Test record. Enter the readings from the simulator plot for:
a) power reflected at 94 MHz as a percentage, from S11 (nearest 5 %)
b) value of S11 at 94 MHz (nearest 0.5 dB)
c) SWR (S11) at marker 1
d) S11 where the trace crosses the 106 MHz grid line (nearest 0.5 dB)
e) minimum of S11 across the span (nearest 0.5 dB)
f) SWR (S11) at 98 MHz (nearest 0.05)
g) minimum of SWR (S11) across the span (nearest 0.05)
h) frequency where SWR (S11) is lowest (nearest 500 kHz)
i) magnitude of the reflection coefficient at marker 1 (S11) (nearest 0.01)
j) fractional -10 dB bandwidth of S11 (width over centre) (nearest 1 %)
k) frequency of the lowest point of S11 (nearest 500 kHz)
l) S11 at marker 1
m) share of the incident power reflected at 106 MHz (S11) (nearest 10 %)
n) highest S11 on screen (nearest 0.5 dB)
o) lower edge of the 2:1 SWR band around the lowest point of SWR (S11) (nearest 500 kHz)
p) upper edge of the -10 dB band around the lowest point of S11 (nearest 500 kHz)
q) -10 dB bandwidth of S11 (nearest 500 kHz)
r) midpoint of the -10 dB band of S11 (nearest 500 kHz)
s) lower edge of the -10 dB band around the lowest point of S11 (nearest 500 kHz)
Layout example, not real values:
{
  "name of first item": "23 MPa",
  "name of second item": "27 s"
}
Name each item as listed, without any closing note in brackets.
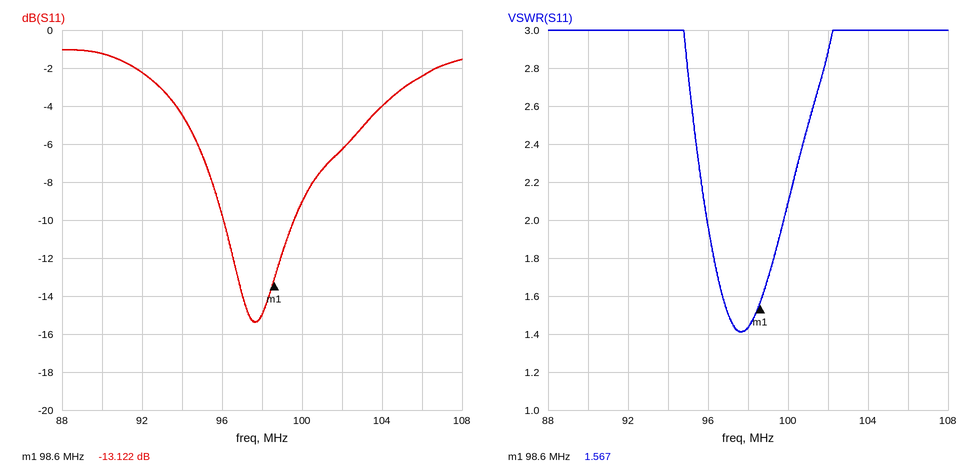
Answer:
{
  "power reflected at 94 MHz as a percentage, from S11": "35 %",
  "value of S11 at 94 MHz": "-4.5 dB",
  "SWR (S11) at marker 1": "1.567",
  "S11 where the trace crosses the 106 MHz grid line": "-2.5 dB",
  "minimum of S11 across the span": "-15.5 dB",
  "SWR (S11) at 98 MHz": "1.45",
  "minimum of SWR (S11) across the span": "1.40",
  "frequency where SWR (S11) is lowest": "97.5 MHz",
  "magnitude of the reflection coefficient at marker 1 (S11)": "0.22",
  "fractional -10 dB bandwidth of S11 (width over centre)": "4 %",
  "frequency of the lowest point of S11": "97.5 MHz",
  "S11 at marker 1": "-13.122 dB",
  "share of the incident power reflected at 106 MHz (S11)": "60 %",
  "highest S11 on screen": "-1.0 dB",
  "lower edge of the 2:1 SWR band around the lowest point of SWR (S11)": "96.0 MHz",
  "upper edge of the -10 dB band around the lowest point of S11": "99.5 MHz",
  "-10 dB bandwidth of S11": "3.5 MHz",
  "midpoint of the -10 dB band of S11": "98.0 MHz",
  "lower edge of the -10 dB band around the lowest point of S11": "96.0 MHz"
}
